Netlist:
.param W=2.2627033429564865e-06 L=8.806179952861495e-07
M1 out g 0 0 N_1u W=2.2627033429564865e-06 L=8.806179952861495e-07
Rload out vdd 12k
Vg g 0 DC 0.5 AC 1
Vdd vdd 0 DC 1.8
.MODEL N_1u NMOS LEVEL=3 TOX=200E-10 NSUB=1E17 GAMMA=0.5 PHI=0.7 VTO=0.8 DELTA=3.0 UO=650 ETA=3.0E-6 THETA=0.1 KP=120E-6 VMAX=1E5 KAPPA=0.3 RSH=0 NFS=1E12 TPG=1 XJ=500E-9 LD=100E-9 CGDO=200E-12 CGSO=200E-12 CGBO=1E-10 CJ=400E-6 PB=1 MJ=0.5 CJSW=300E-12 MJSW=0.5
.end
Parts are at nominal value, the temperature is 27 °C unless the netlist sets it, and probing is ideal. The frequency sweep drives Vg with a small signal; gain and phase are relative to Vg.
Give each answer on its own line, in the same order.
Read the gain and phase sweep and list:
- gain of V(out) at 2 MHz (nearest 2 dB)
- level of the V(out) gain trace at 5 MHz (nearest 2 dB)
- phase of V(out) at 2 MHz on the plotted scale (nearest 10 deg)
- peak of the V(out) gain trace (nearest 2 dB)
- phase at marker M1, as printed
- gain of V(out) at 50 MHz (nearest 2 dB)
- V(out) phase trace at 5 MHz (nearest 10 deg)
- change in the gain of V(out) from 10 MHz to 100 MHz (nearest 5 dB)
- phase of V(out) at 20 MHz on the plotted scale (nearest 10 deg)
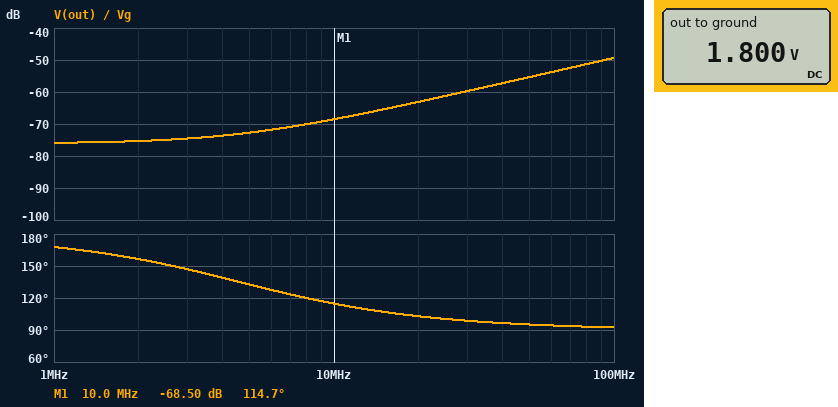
-76 dB
-72 dB
160 deg
-50 dB
114.7 deg
-56 dB
130 deg
20 dB
100 deg
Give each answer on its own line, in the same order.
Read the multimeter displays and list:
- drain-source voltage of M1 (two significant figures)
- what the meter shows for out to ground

1.8 V
1.800 V
